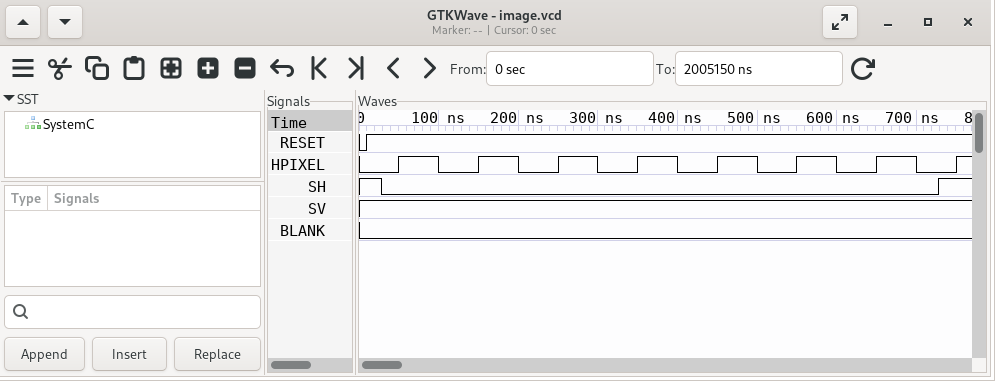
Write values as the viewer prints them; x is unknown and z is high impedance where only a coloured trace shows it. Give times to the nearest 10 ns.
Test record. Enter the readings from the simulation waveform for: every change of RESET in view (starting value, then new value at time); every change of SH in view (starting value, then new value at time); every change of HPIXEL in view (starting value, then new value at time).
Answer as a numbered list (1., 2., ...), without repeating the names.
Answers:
1. 0, 1 at 10 ns
2. 1, 0 at 30 ns, 1 at 730 ns
3. 0, 1 at 50 ns, 0 at 100 ns, 1 at 150 ns, 0 at 200 ns, 1 at 250 ns, 0 at 300 ns, 1 at 350 ns, 0 at 400 ns, 1 at 450 ns, 0 at 500 ns, 1 at 550 ns, 0 at 600 ns, 1 at 650 ns, 0 at 700 ns, 1 at 750 ns
